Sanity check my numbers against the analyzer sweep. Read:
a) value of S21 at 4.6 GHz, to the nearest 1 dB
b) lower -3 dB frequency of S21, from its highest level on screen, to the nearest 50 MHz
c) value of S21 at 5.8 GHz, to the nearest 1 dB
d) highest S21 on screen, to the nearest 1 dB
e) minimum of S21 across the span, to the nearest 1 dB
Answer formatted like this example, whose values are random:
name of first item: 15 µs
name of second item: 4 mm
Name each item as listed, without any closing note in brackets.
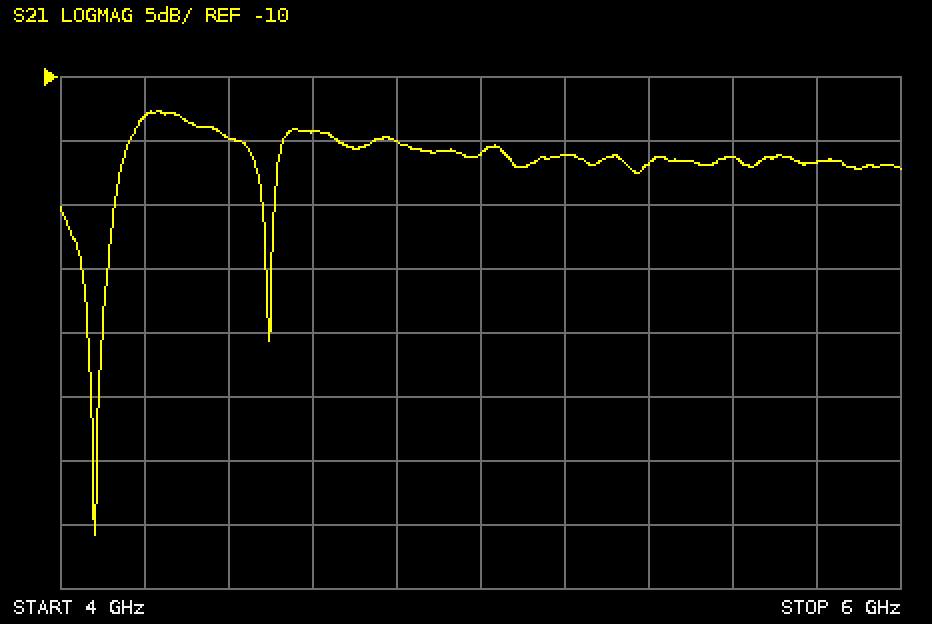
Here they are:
value of S21 at 4.6 GHz, to the nearest 1 dB: -14 dB
lower -3 dB frequency of S21, from its highest level on screen, to the nearest 50 MHz: 4.15 GHz
value of S21 at 5.8 GHz, to the nearest 1 dB: -17 dB
highest S21 on screen, to the nearest 1 dB: -13 dB
minimum of S21 across the span, to the nearest 1 dB: -46 dB
